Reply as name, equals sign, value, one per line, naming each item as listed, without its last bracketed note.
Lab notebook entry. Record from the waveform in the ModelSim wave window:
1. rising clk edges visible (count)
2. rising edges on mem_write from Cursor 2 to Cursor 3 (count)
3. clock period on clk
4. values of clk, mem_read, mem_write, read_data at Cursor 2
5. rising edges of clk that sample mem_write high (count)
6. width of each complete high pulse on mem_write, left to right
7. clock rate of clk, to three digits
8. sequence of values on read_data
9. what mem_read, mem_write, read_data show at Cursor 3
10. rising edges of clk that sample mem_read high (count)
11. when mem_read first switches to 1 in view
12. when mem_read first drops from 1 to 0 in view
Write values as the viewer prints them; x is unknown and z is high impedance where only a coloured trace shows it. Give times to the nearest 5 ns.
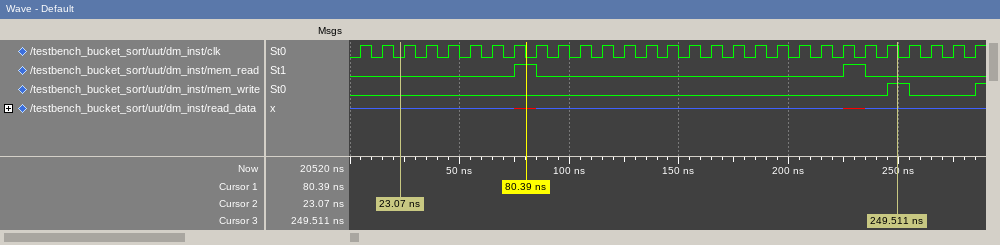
rising clk edges visible = 29
rising edges on mem_write from Cursor 2 to Cursor 3 = 1
clock period on clk = 10 ns
values of clk, mem_read, mem_write, read_data at Cursor 2 = clk=0, mem_read=0, mem_write=0, read_data=z
rising edges of clk that sample mem_write high = 1
width of each complete high pulse on mem_write, left to right = 10 ns
clock rate of clk, to three digits = 100 MHz
sequence of values on read_data = z, x, z, x, z
what mem_read, mem_write, read_data show at Cursor 3 = mem_read=0, mem_write=1, read_data=z
rising edges of clk that sample mem_read high = 2
when mem_read first switches to 1 in view = 75 ns
when mem_read first drops from 1 to 0 in view = 85 ns
